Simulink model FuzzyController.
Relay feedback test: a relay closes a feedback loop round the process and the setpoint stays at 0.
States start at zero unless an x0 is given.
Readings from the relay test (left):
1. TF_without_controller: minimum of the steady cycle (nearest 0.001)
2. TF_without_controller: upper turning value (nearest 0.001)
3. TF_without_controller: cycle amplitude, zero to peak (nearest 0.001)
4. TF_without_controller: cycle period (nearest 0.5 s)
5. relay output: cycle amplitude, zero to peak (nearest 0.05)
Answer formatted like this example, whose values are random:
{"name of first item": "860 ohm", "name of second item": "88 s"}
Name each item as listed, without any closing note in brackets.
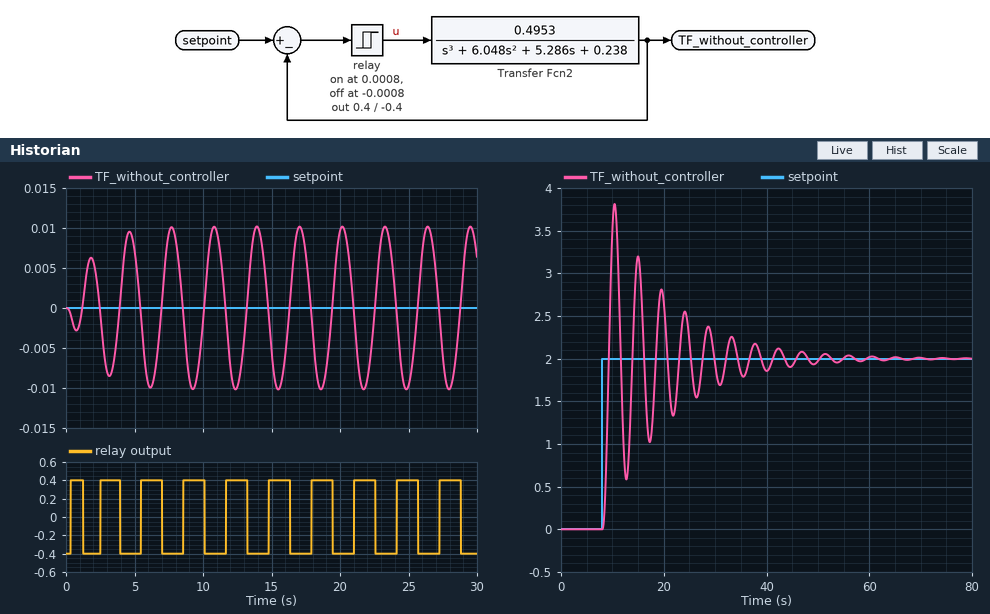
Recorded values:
{"TF_without_controller: minimum of the steady cycle": "-0.010", "TF_without_controller: upper turning value": "0.010", "TF_without_controller: cycle amplitude, zero to peak": "0.010", "TF_without_controller: cycle period": "3.0 s", "relay output: cycle amplitude, zero to peak": "0.40"}
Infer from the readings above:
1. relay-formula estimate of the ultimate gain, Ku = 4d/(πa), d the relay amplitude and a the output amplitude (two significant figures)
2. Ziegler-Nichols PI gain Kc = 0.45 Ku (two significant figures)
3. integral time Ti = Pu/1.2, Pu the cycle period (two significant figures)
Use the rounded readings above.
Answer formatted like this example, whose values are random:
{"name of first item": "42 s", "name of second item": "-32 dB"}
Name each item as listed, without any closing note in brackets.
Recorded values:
{"relay-formula estimate of the ultimate gain, Ku = 4d/(πa), d the relay amplitude and a the output amplitude": "51", "Ziegler-Nichols PI gain Kc = 0.45 Ku": "23", "integral time Ti = Pu/1.2, Pu the cycle period": "2.5 s"}
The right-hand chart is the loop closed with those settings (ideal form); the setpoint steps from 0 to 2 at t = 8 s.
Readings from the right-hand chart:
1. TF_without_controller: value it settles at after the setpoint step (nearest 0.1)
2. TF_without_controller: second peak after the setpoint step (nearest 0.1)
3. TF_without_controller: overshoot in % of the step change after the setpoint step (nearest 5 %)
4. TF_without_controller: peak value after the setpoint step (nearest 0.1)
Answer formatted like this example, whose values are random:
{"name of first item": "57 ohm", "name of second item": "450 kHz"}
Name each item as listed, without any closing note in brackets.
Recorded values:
{"TF_without_controller: value it settles at after the setpoint step": "2.0", "TF_without_controller: second peak after the setpoint step": "3.2", "TF_without_controller: overshoot in % of the step change after the setpoint step": "90 %", "TF_without_controller: peak value after the setpoint step": "3.8"}
